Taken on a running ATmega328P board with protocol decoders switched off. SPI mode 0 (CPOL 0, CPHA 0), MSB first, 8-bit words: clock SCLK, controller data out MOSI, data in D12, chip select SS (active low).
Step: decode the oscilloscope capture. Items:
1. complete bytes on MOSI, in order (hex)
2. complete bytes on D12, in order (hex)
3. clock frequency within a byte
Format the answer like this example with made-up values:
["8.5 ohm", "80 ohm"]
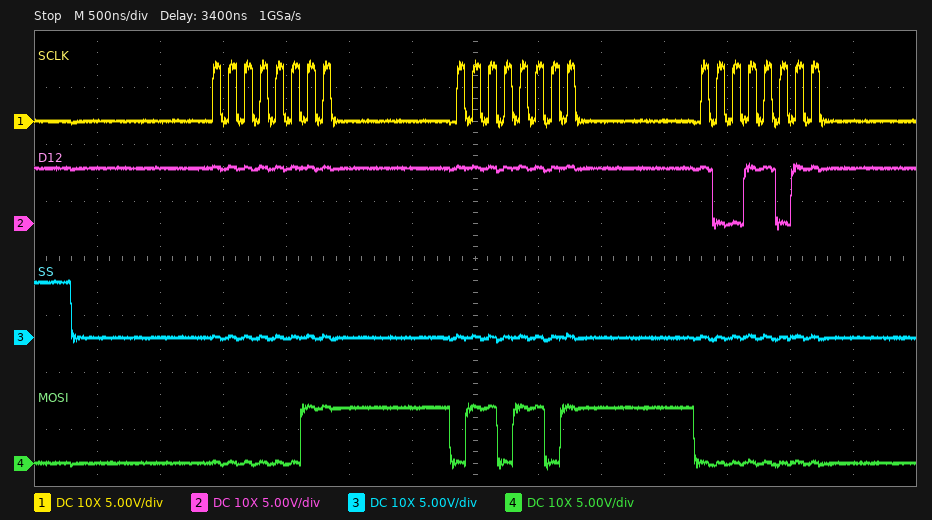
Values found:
["03 6D 00", "FF FF 9B", "8 MHz"]
